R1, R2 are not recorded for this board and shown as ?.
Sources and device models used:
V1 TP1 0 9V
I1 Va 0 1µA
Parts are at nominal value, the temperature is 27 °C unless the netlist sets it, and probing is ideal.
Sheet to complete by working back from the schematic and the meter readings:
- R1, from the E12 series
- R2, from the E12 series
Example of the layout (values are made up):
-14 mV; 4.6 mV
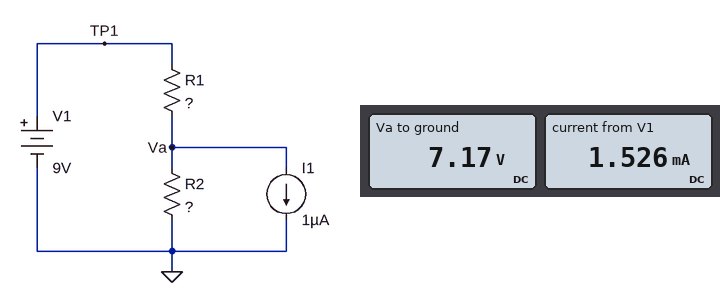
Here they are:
1.2 kΩ; 4.7 kΩ
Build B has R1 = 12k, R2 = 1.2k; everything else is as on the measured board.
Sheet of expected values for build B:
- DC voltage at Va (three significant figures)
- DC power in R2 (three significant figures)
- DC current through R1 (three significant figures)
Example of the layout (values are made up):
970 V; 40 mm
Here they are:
817 mV; 556 µW; 682 µA
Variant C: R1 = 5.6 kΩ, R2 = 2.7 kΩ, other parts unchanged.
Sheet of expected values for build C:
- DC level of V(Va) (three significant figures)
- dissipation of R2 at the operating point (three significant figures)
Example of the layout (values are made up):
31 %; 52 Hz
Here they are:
2.93 V; 3.17 mW
